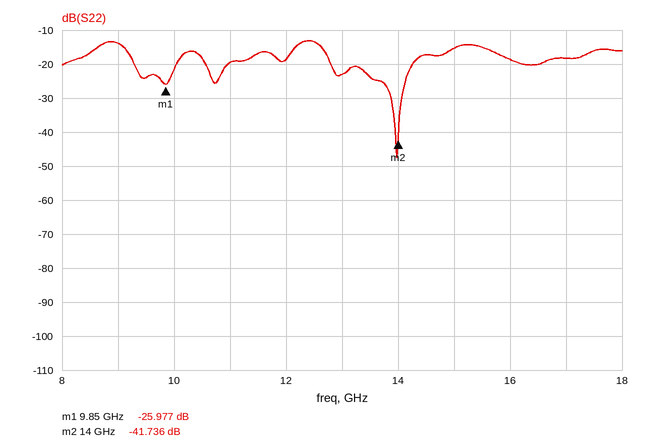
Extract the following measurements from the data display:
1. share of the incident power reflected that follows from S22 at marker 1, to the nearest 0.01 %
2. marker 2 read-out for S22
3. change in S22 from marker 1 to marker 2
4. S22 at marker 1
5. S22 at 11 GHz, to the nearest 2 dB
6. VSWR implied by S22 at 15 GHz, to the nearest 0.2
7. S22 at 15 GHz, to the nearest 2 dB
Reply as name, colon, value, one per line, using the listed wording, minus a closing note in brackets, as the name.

share of the incident power reflected that follows from S22 at marker 1, to the nearest 0.01 %: 0.25 %
marker 2 read-out for S22: -41.736 dB
change in S22 from marker 1 to marker 2: -15.759 dB
S22 at marker 1: -25.977 dB
S22 at 11 GHz, to the nearest 2 dB: -20 dB
VSWR implied by S22 at 15 GHz, to the nearest 0.2: 1.4
S22 at 15 GHz, to the nearest 2 dB: -16 dB
